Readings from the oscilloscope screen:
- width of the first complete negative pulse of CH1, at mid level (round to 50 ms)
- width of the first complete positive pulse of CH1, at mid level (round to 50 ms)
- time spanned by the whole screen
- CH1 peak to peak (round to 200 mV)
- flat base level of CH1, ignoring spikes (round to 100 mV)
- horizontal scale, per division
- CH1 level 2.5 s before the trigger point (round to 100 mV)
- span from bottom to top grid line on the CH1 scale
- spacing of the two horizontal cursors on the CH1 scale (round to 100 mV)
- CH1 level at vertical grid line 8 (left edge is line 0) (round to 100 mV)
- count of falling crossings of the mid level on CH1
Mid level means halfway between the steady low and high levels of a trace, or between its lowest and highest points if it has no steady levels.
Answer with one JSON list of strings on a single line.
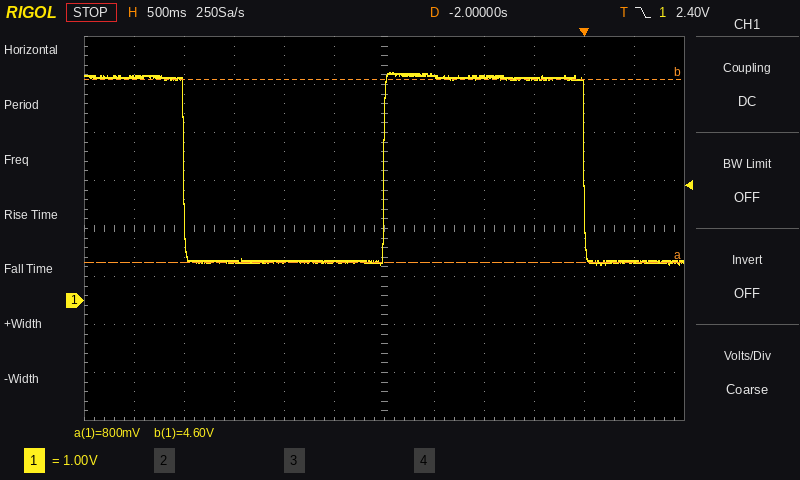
["2.00 s", "2.00 s", "6 s", "4.0 V", "800 mV", "500 ms", "800 mV", "8 V", "3.8 V", "4.7 V", "2"]
